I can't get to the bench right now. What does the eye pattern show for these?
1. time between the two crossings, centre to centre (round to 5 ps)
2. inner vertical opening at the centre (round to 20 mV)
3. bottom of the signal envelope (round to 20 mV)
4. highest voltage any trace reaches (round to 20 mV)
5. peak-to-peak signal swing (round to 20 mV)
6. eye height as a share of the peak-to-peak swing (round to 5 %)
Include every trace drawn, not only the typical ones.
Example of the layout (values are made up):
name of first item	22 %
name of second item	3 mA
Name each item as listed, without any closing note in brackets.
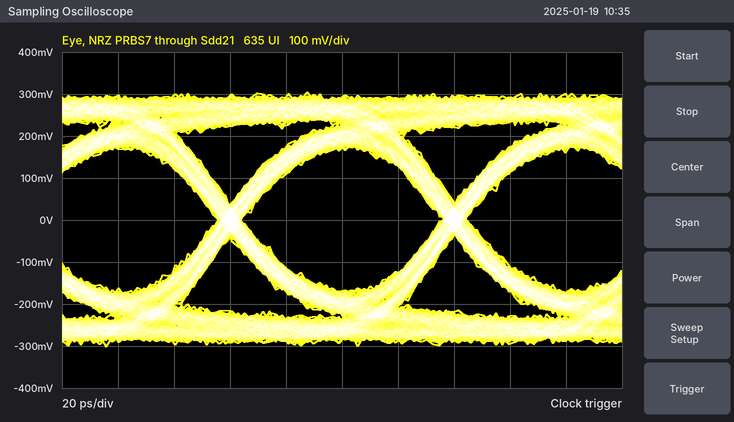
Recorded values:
time between the two crossings, centre to centre	80 ps
inner vertical opening at the centre	340 mV
bottom of the signal envelope	-300 mV
highest voltage any trace reaches	300 mV
peak-to-peak signal swing	600 mV
eye height as a share of the peak-to-peak swing	55 %
